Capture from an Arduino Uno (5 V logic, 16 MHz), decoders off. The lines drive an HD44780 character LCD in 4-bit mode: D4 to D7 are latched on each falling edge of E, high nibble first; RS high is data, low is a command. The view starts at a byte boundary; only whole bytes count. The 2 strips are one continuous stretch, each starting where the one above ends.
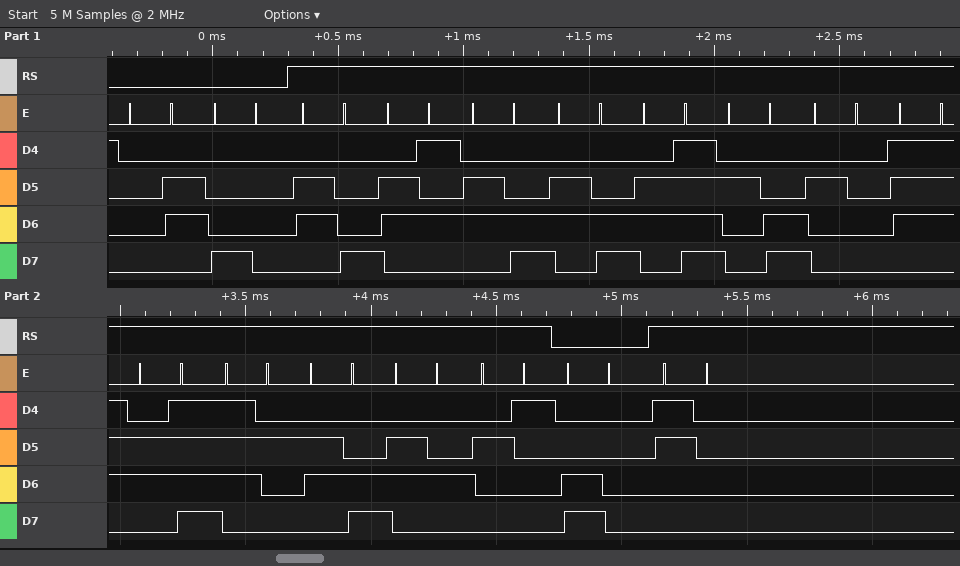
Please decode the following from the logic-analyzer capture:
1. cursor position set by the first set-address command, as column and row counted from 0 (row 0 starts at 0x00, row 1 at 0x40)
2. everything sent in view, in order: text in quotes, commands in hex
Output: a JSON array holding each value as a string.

["column 0, row 0", "0x06 0x80 \"hello, world!\" 0xC0 \"0\""]
